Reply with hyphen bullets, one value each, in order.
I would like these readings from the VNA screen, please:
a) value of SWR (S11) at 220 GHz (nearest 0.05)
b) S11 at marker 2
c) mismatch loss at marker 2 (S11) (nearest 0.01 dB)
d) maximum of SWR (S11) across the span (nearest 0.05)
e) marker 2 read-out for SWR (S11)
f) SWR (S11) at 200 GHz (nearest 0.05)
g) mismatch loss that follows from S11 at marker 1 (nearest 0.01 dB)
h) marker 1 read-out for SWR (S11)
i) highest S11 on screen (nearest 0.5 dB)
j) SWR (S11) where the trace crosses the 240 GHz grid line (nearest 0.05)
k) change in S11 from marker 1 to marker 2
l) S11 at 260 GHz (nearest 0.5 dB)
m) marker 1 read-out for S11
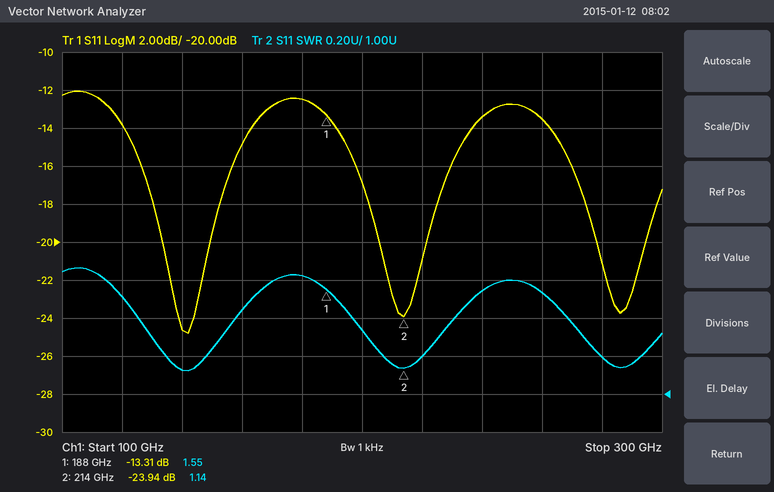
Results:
- 1.20
- -23.94 dB
- 0.02 dB
- 1.65
- 1.14
- 1.35
- 0.21 dB
- 1.55
- -12.0 dB
- 1.55
- -10.63 dB
- -13.5 dB
- -13.31 dB
